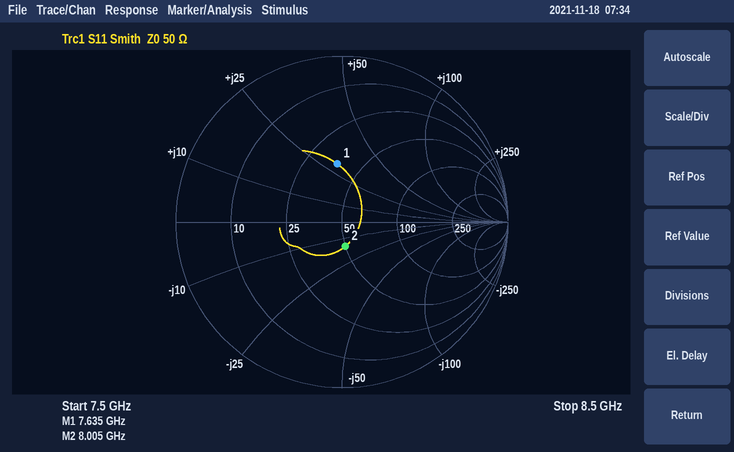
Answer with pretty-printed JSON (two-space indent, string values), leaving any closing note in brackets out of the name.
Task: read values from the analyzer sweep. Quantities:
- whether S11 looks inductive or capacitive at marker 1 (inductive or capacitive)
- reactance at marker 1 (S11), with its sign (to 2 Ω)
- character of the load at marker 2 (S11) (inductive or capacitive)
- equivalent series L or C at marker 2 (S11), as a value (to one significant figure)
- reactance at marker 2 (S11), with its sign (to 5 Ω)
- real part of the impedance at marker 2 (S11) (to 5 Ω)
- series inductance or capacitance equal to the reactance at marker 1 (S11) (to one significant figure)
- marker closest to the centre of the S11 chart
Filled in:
{
  "whether S11 looks inductive or capacitive at marker 1": "inductive",
  "reactance at marker 1 (S11), with its sign": "+30 Ω",
  "character of the load at marker 2 (S11)": "capacitive",
  "equivalent series L or C at marker 2 (S11), as a value": "1 pF",
  "reactance at marker 2 (S11), with its sign": "-15 Ω",
  "real part of the impedance at marker 2 (S11)": "50 Ω",
  "series inductance or capacitance equal to the reactance at marker 1 (S11)": "600 pH",
  "marker closest to the centre of the S11 chart": "marker 2"
}
